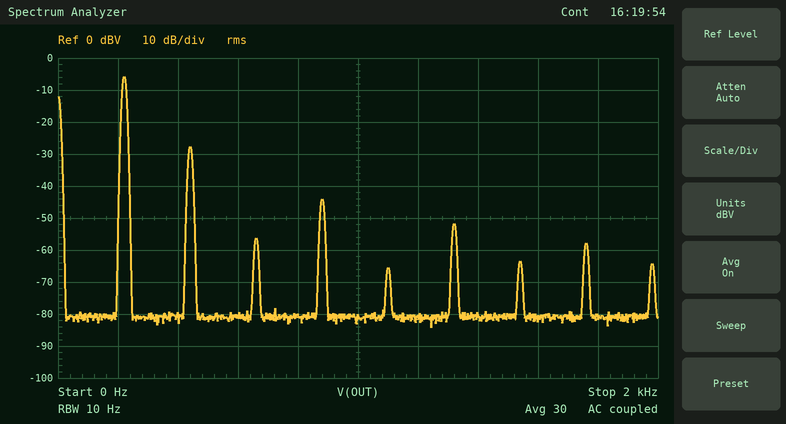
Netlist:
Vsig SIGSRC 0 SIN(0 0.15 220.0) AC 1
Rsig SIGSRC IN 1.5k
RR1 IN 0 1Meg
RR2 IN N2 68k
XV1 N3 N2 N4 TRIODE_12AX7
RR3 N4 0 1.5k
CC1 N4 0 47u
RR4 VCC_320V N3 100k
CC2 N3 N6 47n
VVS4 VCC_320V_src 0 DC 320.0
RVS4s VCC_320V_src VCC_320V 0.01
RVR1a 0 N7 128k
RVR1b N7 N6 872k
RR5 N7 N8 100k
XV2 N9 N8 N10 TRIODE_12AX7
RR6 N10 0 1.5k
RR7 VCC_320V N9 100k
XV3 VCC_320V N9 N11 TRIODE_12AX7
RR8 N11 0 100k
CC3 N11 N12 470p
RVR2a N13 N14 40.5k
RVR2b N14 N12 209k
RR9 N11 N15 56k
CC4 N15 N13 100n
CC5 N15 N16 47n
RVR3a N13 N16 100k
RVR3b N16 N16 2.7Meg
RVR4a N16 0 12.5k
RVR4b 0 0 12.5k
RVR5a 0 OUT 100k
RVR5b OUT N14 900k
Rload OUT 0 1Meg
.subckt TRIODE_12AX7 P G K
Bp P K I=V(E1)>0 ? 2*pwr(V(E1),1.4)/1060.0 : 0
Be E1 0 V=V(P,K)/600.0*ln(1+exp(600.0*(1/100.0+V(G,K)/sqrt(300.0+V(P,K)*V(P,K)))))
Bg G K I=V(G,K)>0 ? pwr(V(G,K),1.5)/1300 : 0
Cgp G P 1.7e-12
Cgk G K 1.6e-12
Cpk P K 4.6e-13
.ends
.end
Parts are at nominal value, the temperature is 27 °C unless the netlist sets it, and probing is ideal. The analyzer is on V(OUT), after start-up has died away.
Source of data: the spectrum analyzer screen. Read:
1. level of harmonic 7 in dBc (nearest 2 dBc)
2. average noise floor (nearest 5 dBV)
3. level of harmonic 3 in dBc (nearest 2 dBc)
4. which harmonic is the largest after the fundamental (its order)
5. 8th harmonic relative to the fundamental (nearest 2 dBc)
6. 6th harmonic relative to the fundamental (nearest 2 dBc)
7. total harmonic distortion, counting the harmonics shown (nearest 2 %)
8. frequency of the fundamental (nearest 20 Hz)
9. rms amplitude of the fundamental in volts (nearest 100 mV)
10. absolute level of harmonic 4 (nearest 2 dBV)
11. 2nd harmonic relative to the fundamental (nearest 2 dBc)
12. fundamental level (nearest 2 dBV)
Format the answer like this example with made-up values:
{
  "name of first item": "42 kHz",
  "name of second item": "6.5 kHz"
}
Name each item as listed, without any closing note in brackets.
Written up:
{
  "level of harmonic 7 in dBc": "-58 dBc",
  "average noise floor": "-80 dBV",
  "level of harmonic 3 in dBc": "-50 dBc",
  "which harmonic is the largest after the fundamental": "2",
  "8th harmonic relative to the fundamental": "-52 dBc",
  "6th harmonic relative to the fundamental": "-46 dBc",
  "total harmonic distortion, counting the harmonics shown": "8 %",
  "frequency of the fundamental": "220 Hz",
  "rms amplitude of the fundamental in volts": "500 mV",
  "absolute level of harmonic 4": "-44 dBV",
  "2nd harmonic relative to the fundamental": "-22 dBc",
  "fundamental level": "-6 dBV"
}
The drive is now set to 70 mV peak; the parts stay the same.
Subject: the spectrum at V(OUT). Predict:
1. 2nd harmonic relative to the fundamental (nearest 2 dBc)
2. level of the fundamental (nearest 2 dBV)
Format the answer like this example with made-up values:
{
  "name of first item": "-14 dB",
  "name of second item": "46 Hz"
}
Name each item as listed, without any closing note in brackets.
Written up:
{
  "2nd harmonic relative to the fundamental": "-24 dBc",
  "level of the fundamental": "-12 dBV"
}
